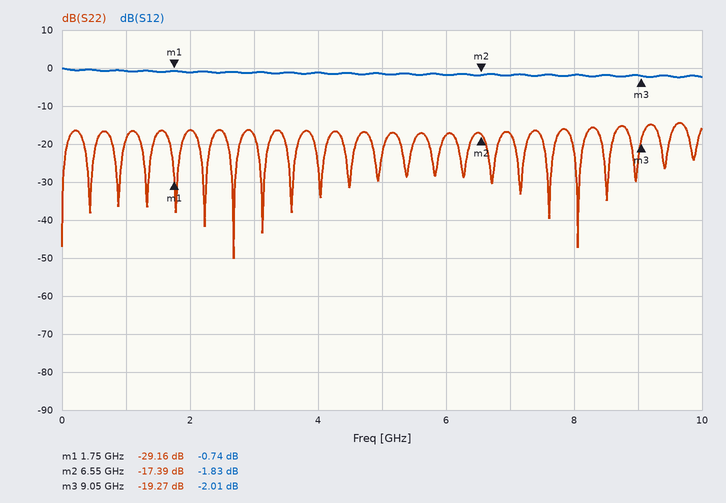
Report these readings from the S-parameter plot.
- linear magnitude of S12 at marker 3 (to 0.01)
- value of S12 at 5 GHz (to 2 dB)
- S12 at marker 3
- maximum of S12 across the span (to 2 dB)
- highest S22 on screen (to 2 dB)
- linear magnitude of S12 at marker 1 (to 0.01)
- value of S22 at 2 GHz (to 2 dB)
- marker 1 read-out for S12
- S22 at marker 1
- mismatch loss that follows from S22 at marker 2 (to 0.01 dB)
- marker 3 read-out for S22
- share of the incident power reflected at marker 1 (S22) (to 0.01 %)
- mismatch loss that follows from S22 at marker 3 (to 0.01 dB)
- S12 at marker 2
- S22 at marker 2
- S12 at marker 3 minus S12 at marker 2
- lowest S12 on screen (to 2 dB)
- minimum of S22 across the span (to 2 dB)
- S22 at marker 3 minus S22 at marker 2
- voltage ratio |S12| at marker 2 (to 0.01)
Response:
0.79
-2 dB
-2.01 dB
0 dB
-14 dB
0.92
-16 dB
-0.74 dB
-29.16 dB
0.08 dB
-19.27 dB
0.12 %
0.05 dB
-1.83 dB
-17.39 dB
-0.18 dB
-2 dB
-50 dB
-1.88 dB
0.81
